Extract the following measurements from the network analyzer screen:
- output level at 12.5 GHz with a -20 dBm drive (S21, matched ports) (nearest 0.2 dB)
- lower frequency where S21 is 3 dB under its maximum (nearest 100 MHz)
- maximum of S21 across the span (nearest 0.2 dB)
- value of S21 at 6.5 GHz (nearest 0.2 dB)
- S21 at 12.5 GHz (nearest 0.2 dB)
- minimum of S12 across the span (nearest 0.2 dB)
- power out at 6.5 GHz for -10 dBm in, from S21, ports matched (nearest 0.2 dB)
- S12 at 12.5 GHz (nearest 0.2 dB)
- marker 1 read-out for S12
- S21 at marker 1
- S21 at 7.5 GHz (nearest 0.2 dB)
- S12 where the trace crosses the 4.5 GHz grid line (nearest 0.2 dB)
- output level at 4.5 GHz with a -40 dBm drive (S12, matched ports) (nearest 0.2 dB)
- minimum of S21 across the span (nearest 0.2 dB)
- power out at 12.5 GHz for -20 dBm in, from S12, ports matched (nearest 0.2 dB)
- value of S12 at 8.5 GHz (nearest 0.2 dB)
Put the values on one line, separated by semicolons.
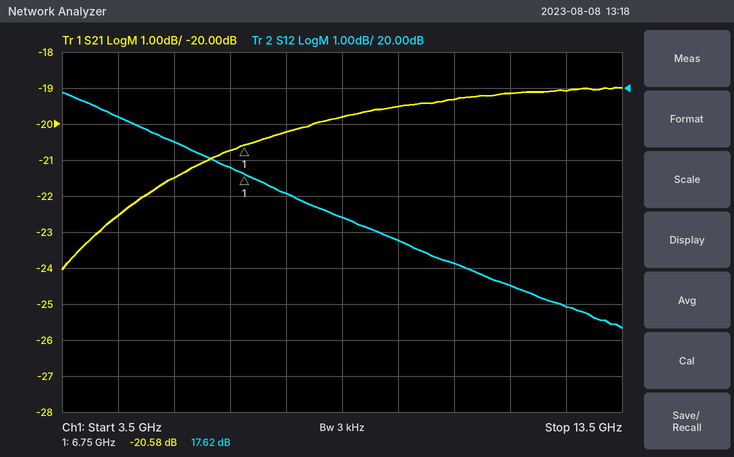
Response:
-39.0 dBm; 5.0 GHz; -19.0 dB; -20.8 dB; -19.0 dB; 13.4 dB; -30.8 dBm; 14.0 dB; 17.62 dB; -20.58 dB; -20.2 dB; 19.2 dB; -20.8 dBm; -24.0 dB; -6.0 dBm; 16.4 dB
